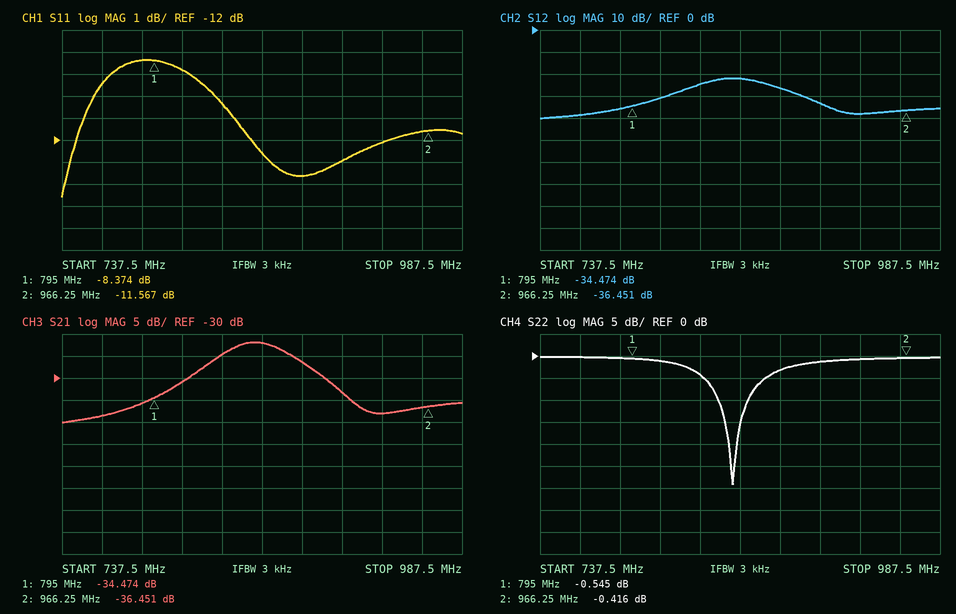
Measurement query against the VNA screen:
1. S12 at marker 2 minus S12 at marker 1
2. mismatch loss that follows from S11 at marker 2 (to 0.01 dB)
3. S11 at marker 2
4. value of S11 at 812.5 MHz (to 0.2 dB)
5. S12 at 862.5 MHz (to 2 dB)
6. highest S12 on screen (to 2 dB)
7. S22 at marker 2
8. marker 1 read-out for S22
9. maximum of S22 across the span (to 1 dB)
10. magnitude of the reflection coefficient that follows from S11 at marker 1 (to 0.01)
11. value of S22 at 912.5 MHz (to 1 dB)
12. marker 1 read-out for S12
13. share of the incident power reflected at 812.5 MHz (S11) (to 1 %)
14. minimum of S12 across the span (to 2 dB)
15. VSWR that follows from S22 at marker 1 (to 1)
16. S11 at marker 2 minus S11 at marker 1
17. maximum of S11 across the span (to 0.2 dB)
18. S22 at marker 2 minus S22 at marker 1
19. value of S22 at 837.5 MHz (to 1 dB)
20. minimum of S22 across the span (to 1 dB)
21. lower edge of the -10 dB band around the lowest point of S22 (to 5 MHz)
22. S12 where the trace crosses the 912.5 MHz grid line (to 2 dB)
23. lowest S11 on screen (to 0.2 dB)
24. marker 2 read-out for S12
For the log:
-1.977 dB
0.31 dB
-11.567 dB
-8.8 dB
-22 dB
-22 dB
-0.416 dB
-0.545 dB
0 dB
0.38
-1 dB
-34.474 dB
13 %
-40 dB
32
-3.193 dB
-8.4 dB
0.129 dB
-4 dB
-29 dB
850 MHz
-34 dB
-14.6 dB
-36.451 dB
